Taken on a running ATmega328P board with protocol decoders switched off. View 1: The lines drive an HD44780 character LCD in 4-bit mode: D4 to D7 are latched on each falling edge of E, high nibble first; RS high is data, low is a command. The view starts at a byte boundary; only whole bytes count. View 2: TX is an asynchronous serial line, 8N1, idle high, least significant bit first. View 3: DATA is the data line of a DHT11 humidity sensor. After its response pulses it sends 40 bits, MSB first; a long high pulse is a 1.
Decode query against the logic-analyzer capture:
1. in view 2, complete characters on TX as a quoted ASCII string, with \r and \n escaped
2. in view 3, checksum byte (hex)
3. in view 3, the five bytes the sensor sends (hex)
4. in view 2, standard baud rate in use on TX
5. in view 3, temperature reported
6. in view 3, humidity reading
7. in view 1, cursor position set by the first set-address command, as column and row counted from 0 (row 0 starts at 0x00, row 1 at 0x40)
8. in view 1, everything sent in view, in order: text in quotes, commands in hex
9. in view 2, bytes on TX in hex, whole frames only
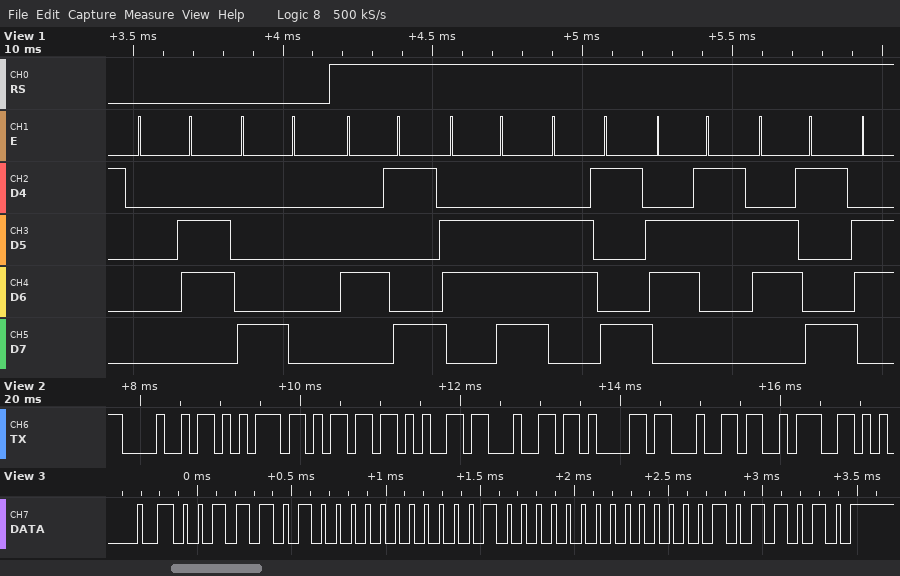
"Humedad:"
0x5A
3A 00 20 00 5A
9600 baud
32.0 °C
58 %
column 0, row 0
0x06 0x80 "Inici"
48 75 6D 65 64 61 64 3A
